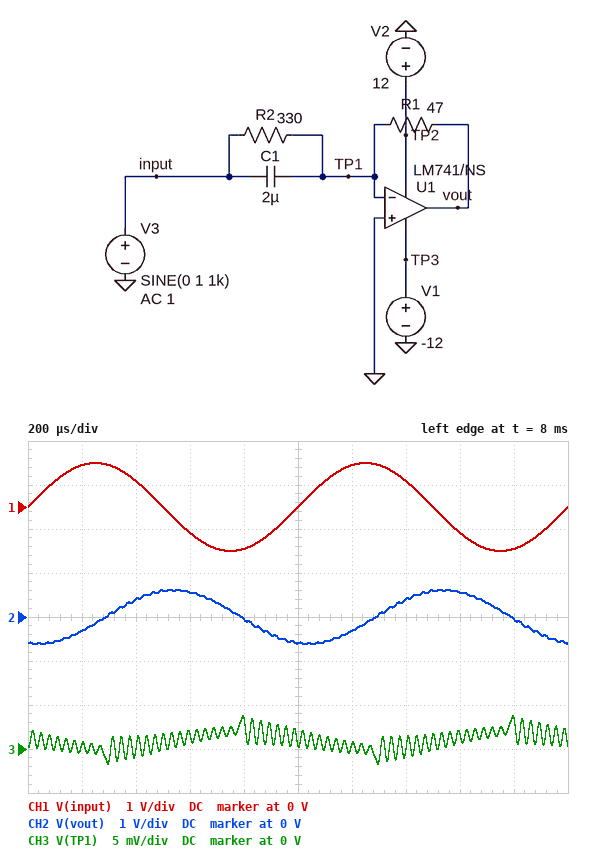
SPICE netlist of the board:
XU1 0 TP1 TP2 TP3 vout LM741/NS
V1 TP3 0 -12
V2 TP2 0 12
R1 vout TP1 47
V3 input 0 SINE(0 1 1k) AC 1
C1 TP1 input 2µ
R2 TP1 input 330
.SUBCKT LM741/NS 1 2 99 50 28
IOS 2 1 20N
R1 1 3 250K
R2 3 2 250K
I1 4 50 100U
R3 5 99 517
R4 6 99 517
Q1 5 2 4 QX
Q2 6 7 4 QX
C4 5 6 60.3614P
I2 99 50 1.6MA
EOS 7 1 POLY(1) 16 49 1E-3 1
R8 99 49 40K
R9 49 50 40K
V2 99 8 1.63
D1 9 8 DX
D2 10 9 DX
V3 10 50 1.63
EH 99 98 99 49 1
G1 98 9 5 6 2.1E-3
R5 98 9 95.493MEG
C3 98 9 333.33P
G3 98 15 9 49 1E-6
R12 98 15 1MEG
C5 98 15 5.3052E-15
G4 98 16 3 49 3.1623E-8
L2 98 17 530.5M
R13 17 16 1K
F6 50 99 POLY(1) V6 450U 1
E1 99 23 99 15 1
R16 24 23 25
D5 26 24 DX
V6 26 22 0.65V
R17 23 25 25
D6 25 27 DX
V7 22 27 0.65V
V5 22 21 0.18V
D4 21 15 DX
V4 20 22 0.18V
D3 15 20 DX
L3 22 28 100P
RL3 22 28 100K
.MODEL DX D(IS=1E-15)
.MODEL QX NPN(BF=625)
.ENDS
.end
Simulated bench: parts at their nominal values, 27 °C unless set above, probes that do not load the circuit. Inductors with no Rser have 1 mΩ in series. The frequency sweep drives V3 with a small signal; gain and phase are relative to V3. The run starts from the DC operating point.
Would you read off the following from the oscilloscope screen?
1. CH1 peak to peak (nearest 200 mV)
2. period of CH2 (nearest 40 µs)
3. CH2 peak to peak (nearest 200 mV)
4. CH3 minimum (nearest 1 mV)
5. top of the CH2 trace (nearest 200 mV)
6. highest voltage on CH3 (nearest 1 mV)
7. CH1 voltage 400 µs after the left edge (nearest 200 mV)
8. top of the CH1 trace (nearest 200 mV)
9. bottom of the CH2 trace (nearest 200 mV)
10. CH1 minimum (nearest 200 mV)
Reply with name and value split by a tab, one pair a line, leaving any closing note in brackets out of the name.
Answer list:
CH1 peak to peak	2.0 V
period of CH2	1.00 ms
CH2 peak to peak	1.2 V
CH3 minimum	-2 mV
top of the CH2 trace	600 mV
highest voltage on CH3	4 mV
CH1 voltage 400 µs after the left edge	600 mV
top of the CH1 trace	1.0 V
bottom of the CH2 trace	-600 mV
CH1 minimum	-1.0 V
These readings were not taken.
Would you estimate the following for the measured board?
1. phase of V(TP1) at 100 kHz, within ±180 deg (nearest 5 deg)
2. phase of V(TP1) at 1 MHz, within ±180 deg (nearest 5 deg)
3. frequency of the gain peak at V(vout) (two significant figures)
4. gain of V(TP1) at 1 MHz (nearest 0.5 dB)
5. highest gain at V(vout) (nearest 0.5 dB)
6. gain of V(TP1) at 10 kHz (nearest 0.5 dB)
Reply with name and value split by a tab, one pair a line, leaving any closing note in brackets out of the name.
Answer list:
phase of V(TP1) at 100 kHz, within ±180 deg	0 deg
phase of V(TP1) at 1 MHz, within ±180 deg	0 deg
frequency of the gain peak at V(vout)	19 kHz
gain of V(TP1) at 1 MHz	0 dB
highest gain at V(vout)	53.5 dB
gain of V(TP1) at 10 kHz	-8.0 dB
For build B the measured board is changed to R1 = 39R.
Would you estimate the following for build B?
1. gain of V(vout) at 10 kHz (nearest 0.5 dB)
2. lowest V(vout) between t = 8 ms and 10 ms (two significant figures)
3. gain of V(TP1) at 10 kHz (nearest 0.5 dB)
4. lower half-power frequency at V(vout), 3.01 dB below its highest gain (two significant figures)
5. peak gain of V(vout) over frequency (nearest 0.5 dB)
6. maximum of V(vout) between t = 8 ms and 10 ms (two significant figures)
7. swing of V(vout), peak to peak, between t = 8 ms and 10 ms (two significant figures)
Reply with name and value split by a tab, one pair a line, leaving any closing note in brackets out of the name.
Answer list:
gain of V(vout) at 10 kHz	16.5 dB
lowest V(vout) between t = 8 ms and 10 ms	-520 mV
gain of V(TP1) at 10 kHz	-8.5 dB
lower half-power frequency at V(vout), 3.01 dB below its highest gain	19 kHz
peak gain of V(vout) over frequency	52.0 dB
maximum of V(vout) between t = 8 ms and 10 ms	520 mV
swing of V(vout), peak to peak, between t = 8 ms and 10 ms	1.0 V
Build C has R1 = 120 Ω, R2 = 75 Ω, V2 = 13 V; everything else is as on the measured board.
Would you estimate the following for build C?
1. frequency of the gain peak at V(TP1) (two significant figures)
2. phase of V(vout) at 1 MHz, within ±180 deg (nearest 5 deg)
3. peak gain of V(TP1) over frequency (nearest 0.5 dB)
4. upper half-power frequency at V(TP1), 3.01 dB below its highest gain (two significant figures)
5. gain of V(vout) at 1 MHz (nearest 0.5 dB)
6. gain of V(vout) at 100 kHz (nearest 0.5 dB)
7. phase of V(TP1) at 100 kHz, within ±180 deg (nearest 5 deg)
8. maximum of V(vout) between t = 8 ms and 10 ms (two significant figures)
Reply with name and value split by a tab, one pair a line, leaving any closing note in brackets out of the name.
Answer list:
frequency of the gain peak at V(TP1)	16 kHz
phase of V(vout) at 1 MHz, within ±180 deg	25 deg
peak gain of V(TP1) over frequency	22.5 dB
upper half-power frequency at V(TP1), 3.01 dB below its highest gain	17 kHz
gain of V(vout) at 1 MHz	-1.5 dB
gain of V(vout) at 100 kHz	12.5 dB
phase of V(TP1) at 100 kHz, within ±180 deg	0 deg
maximum of V(vout) between t = 8 ms and 10 ms	2.2 V
